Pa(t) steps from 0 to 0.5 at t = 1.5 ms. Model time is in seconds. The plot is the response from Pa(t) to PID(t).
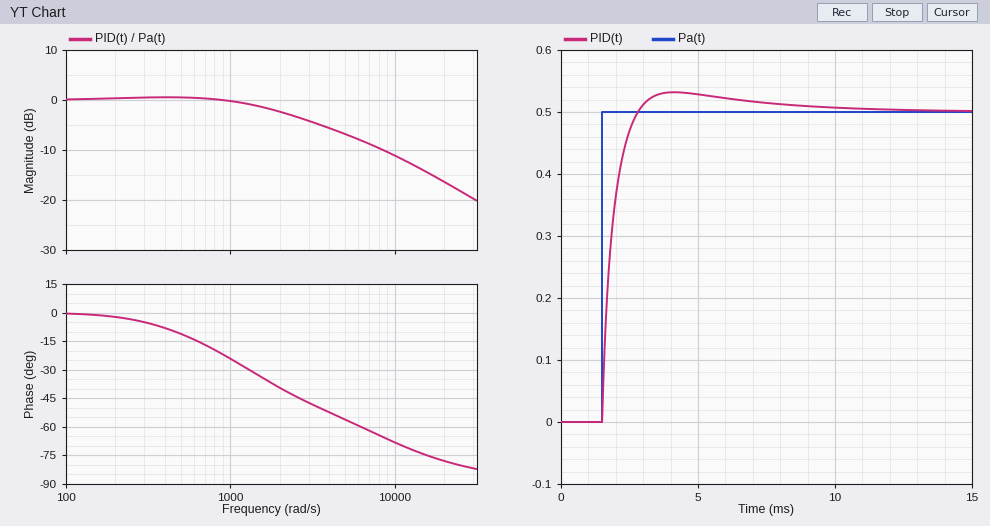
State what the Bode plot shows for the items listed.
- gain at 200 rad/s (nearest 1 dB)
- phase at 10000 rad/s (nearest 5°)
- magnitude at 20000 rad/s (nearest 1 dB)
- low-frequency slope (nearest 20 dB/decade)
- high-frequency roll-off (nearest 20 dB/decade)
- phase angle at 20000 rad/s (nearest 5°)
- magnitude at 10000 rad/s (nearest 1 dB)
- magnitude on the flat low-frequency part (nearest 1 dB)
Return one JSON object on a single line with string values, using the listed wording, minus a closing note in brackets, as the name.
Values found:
{"gain at 200 rad/s": "0 dB", "phase at 10000 rad/s": "-70°", "magnitude at 20000 rad/s": "-16 dB", "low-frequency slope": "0 dB/decade", "high-frequency roll-off": "-20 dB/decade", "phase angle at 20000 rad/s": "-80°", "magnitude at 10000 rad/s": "-11 dB", "magnitude on the flat low-frequency part": "0 dB"}
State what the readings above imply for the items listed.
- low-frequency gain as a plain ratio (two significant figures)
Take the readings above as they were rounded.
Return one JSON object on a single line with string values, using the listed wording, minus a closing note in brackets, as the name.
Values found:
{"low-frequency gain as a plain ratio": "1.0"}
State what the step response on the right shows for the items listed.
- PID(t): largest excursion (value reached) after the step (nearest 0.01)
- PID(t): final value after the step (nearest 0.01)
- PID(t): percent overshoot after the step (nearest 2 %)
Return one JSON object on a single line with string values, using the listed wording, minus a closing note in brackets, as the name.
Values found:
{"PID(t): largest excursion (value reached) after the step": "0.53", "PID(t): final value after the step": "0.50", "PID(t): percent overshoot after the step": "6 %"}
